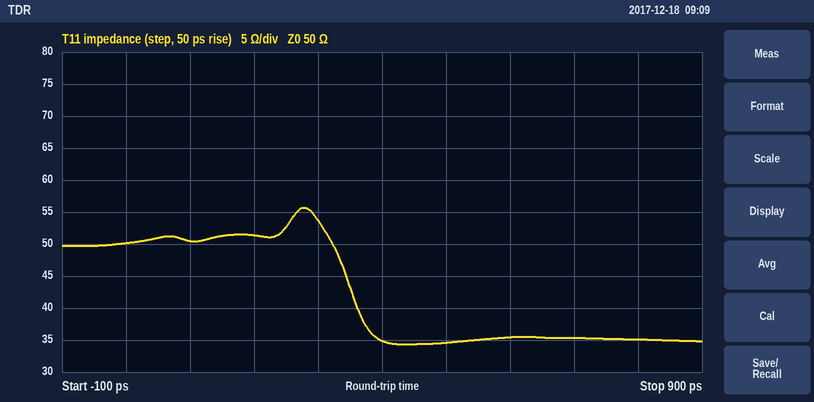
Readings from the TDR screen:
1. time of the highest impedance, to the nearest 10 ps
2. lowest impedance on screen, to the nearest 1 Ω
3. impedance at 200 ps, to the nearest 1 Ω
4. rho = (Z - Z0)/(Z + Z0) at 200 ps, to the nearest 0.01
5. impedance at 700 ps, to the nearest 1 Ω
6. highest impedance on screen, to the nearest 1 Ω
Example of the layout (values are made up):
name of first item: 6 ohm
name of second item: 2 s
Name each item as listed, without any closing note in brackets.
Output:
time of the highest impedance, to the nearest 10 ps: 280 ps
lowest impedance on screen, to the nearest 1 Ω: 34 Ω
impedance at 200 ps, to the nearest 1 Ω: 51 Ω
rho = (Z - Z0)/(Z + Z0) at 200 ps, to the nearest 0.01: +0.01
impedance at 700 ps, to the nearest 1 Ω: 35 Ω
highest impedance on screen, to the nearest 1 Ω: 56 Ω
